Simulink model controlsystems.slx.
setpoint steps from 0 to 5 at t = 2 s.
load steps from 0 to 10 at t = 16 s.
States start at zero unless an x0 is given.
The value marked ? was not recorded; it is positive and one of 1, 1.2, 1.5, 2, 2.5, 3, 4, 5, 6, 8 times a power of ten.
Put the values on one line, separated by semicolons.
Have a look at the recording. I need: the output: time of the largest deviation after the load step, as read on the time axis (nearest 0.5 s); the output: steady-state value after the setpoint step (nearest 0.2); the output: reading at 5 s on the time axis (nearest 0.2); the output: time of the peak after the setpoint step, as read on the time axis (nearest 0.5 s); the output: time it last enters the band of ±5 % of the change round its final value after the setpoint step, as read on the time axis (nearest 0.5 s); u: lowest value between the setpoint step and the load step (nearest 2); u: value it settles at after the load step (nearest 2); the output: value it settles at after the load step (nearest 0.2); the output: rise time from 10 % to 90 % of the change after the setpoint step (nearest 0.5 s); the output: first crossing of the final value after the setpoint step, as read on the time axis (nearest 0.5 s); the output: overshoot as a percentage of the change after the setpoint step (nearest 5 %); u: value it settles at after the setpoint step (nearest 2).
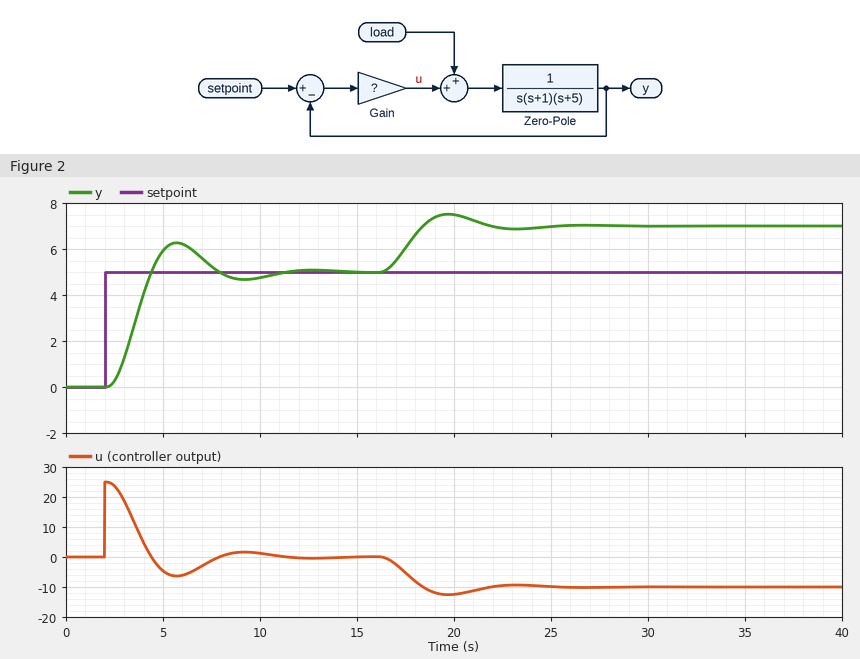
19.5 s; 5.0; 6.0; 5.5 s; 10.0 s; -6; -10; 7.0; 1.5 s; 4.5 s; 25 %; 0
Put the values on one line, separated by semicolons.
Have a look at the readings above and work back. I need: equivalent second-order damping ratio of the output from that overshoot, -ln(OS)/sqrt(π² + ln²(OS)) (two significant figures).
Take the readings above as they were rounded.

0.40
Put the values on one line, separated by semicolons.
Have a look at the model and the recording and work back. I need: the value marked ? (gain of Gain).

5
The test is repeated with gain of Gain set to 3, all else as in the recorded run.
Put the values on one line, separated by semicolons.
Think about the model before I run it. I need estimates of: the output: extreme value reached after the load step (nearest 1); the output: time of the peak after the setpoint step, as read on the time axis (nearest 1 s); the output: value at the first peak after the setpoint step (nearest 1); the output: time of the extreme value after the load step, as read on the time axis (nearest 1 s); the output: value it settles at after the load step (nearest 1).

9; 7 s; 6; 21 s; 8
